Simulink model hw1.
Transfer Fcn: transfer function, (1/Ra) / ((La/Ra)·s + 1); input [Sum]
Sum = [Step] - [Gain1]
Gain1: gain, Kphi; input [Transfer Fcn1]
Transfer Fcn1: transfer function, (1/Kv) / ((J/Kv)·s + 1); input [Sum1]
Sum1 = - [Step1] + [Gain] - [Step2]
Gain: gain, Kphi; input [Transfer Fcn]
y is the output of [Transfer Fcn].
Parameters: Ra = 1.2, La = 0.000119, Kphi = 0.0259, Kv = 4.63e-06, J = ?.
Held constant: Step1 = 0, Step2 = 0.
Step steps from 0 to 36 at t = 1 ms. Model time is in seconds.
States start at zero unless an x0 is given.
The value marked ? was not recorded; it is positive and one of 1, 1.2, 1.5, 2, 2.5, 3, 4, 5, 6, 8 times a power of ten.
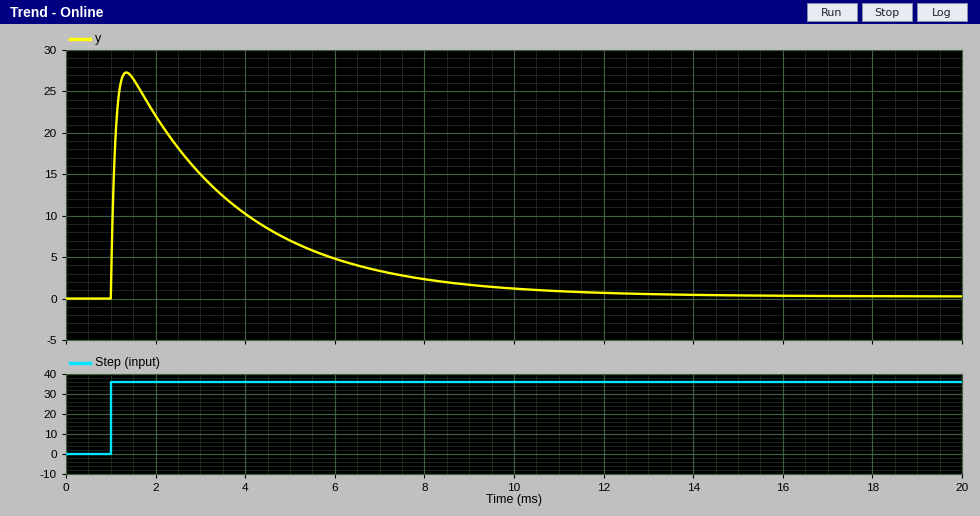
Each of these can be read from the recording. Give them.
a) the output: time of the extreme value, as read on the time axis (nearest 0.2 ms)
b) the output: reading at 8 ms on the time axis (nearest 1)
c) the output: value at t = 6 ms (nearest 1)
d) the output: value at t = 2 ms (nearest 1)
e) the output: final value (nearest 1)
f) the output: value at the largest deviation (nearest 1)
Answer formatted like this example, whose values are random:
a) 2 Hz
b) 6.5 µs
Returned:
a) 1.4 ms
b) 2
c) 5
d) 22
e) 0
f) 27
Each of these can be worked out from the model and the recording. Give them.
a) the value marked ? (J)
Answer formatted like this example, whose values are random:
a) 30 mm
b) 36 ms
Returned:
a) 1.5e-06
